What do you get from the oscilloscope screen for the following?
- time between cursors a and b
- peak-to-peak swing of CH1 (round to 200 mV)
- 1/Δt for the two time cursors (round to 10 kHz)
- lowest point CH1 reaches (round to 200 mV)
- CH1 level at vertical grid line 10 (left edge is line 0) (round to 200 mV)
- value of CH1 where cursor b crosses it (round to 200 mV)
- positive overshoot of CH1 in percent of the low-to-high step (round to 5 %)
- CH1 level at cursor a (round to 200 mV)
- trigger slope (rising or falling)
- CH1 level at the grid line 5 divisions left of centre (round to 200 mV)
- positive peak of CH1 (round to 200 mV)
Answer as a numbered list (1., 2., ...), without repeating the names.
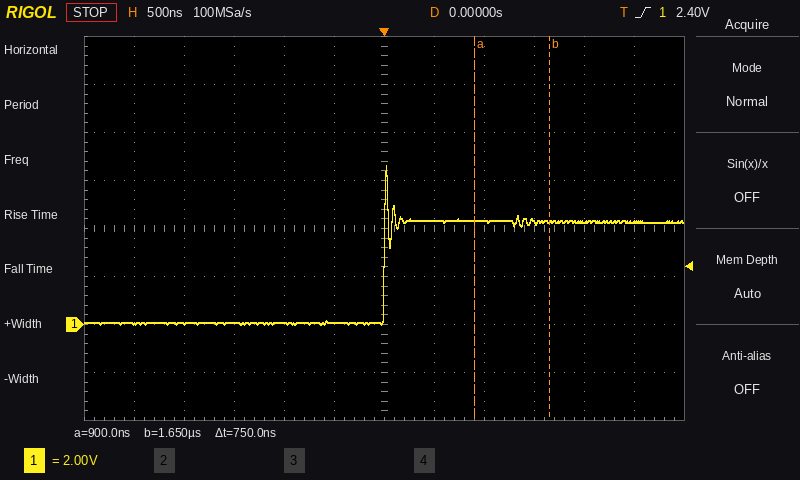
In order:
1. 750 ns
2. 6.6 V
3. 1.33 MHz
4. 0.0 V
5. 4.2 V
6. 4.2 V
7. 55 %
8. 4.4 V
9. rising
10. 0.0 V
11. 6.6 V
